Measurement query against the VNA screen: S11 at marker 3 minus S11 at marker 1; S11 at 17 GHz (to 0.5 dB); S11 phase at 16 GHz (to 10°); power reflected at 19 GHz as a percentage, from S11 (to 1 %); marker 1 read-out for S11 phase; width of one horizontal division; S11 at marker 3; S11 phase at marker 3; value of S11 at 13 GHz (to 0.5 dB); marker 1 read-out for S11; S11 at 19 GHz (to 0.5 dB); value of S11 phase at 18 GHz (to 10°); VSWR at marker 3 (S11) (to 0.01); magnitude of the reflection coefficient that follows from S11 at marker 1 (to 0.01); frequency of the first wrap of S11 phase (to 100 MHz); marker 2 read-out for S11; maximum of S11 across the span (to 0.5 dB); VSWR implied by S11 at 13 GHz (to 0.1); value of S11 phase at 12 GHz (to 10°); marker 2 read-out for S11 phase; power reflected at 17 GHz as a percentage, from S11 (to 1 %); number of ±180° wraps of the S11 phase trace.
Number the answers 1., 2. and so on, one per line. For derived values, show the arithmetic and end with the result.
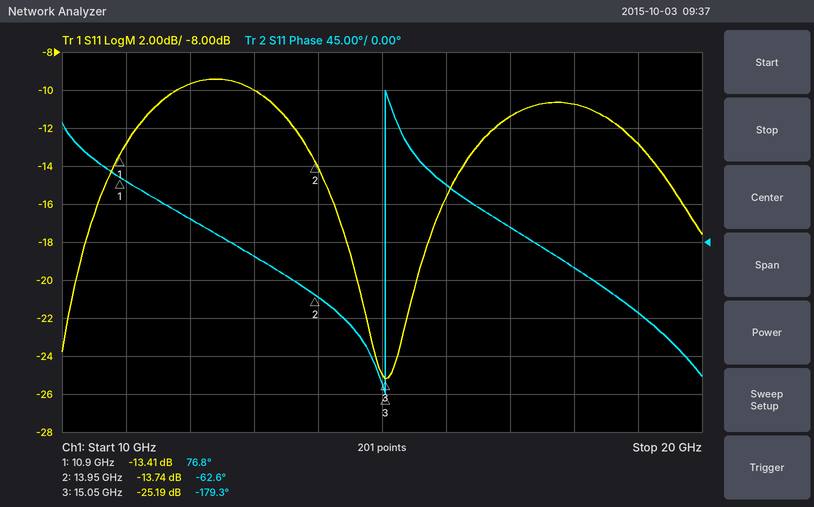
1. -25.19 − (-13.41) = -11.78 dB
2. -11.5 dB
3. 70°
4. 10^(-13/10) ≈ 5 %
5. 76.8°
6. 1 GHz
7. -25.19 dB
8. -179.3°
9. -10.0 dB
10. -13.41 dB
11. -13.0 dB
12. -30°
13. (1 + 0.0550)/(1 − 0.0550) ≈ 1.12
14. 10^(-13.41/20) ≈ 0.21
15. 15.1 GHz
16. -13.74 dB
17. -9.5 dB
18. |Γ| = 10^(-10/20) = 0.3162; VSWR = (1 + 0.3162)/(1 − 0.3162) ≈ 1.9
19. 30°
20. -62.6°
21. 10^(-11.5/10) ≈ 7 %
22. 1
